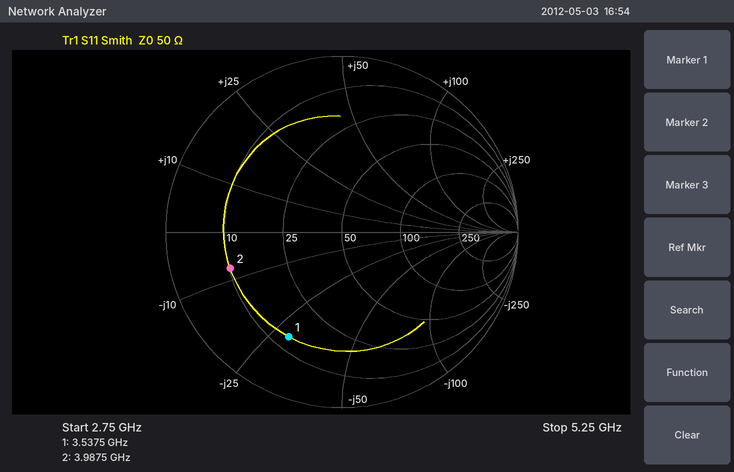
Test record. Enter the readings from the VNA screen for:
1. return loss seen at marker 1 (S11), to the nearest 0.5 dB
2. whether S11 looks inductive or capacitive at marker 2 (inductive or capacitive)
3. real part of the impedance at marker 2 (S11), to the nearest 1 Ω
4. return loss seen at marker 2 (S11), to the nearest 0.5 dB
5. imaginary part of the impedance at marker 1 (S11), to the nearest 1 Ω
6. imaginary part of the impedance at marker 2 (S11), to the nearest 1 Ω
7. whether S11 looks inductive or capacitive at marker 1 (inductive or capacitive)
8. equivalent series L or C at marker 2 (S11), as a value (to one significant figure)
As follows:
3.5 dB
capacitive
10 Ω
3.5 dB
-29 Ω
-8 Ω
capacitive
5 pF
